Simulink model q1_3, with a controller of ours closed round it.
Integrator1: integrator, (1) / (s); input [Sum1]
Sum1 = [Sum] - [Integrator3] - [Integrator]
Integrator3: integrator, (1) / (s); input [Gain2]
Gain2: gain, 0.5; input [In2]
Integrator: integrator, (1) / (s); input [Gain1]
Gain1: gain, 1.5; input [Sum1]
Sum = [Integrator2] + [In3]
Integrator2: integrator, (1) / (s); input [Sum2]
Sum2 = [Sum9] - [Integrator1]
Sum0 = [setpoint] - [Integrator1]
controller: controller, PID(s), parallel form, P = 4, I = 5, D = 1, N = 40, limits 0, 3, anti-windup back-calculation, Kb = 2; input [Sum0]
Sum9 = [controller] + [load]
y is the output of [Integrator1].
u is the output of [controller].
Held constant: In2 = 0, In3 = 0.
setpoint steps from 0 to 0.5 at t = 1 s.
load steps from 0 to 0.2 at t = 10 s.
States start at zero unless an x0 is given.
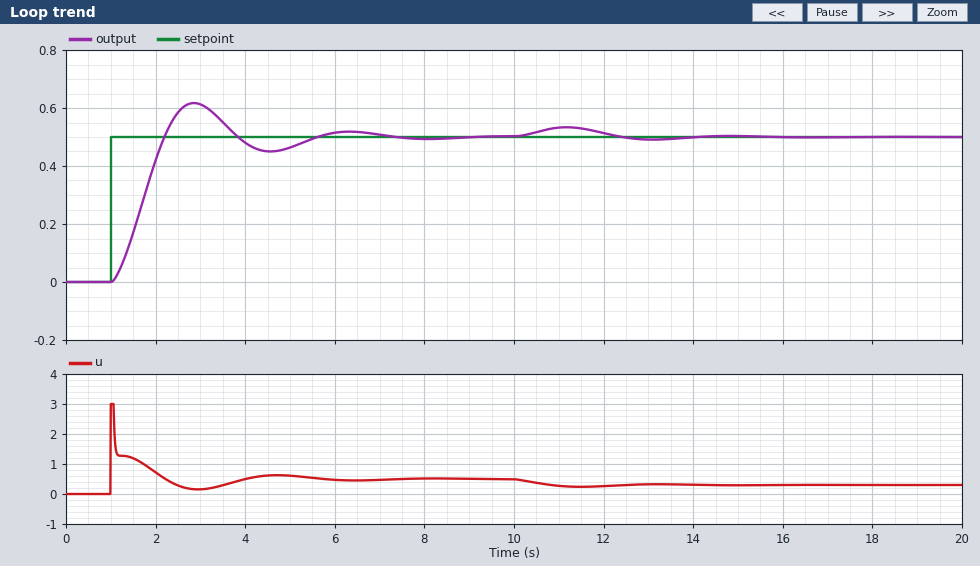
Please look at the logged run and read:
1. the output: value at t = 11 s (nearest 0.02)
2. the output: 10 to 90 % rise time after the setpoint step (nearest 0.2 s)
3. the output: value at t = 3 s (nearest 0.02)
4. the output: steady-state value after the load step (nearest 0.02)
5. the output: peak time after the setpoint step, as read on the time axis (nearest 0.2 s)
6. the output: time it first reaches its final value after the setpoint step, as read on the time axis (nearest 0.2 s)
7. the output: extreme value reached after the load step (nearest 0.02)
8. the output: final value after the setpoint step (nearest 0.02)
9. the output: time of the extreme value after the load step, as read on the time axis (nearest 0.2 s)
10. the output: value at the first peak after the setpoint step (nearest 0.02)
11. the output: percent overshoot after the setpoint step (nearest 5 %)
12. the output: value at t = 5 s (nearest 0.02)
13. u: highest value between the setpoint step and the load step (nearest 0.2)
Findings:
0.54
0.8 s
0.62
0.50
2.8 s
2.2 s
0.54
0.50
11.2 s
0.62
25 %
0.46
3.0
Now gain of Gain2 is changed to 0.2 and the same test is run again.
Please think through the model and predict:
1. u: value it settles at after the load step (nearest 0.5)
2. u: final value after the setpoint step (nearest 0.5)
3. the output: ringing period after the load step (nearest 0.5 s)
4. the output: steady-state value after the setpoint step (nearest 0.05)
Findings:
0.5
0.5
3.5 s
0.50
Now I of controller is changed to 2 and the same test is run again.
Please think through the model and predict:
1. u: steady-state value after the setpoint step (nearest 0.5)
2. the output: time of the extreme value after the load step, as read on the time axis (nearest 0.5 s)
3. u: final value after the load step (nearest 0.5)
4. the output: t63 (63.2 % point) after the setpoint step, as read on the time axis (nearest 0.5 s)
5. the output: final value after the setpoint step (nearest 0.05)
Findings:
0.5
11.5 s
0.5
2.0 s
0.50
